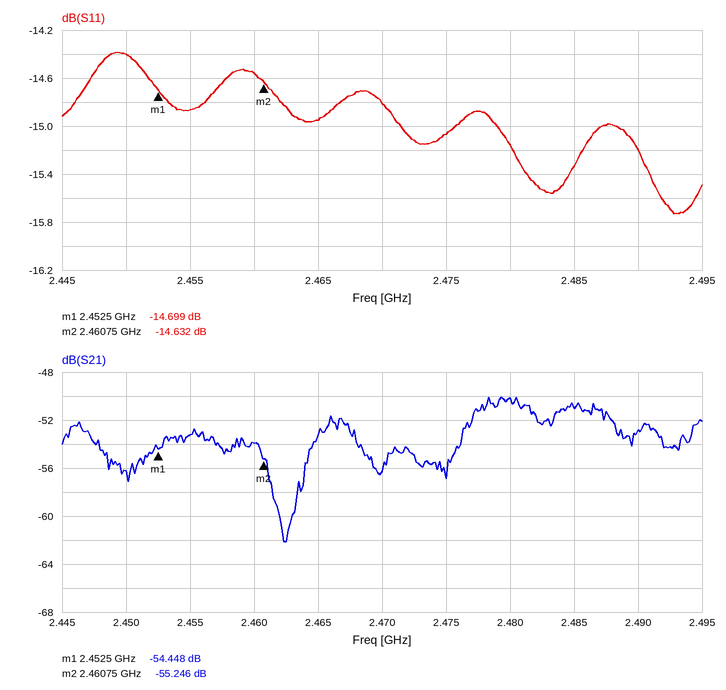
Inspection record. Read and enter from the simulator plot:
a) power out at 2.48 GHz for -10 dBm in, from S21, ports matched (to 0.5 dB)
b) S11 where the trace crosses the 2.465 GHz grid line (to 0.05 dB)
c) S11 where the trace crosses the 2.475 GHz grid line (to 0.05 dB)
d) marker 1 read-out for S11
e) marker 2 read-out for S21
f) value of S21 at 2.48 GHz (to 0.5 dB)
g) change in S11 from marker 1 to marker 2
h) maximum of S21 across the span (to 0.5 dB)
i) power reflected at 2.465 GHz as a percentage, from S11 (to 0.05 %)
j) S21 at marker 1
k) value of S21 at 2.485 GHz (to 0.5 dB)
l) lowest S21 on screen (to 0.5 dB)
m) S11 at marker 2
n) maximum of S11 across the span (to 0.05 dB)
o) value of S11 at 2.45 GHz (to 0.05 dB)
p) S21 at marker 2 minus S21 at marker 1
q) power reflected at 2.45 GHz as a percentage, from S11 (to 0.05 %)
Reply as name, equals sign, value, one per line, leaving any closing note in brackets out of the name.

power out at 2.48 GHz for -10 dBm in, from S21, ports matched = -60.0 dBm
S11 where the trace crosses the 2.465 GHz grid line = -14.95 dB
S11 where the trace crosses the 2.475 GHz grid line = -15.05 dB
marker 1 read-out for S11 = -14.699 dB
marker 2 read-out for S21 = -55.246 dB
value of S21 at 2.48 GHz = -50.0 dB
change in S11 from marker 1 to marker 2 = 0.067 dB
maximum of S21 across the span = -50.0 dB
power reflected at 2.465 GHz as a percentage, from S11 = 3.20 %
S21 at marker 1 = -54.448 dB
value of S21 at 2.485 GHz = -51.0 dB
lowest S21 on screen = -62.0 dB
S11 at marker 2 = -14.632 dB
maximum of S11 across the span = -14.40 dB
value of S11 at 2.45 GHz = -14.40 dB
S21 at marker 2 minus S21 at marker 1 = -0.798 dB
power reflected at 2.45 GHz as a percentage, from S11 = 3.65 %
